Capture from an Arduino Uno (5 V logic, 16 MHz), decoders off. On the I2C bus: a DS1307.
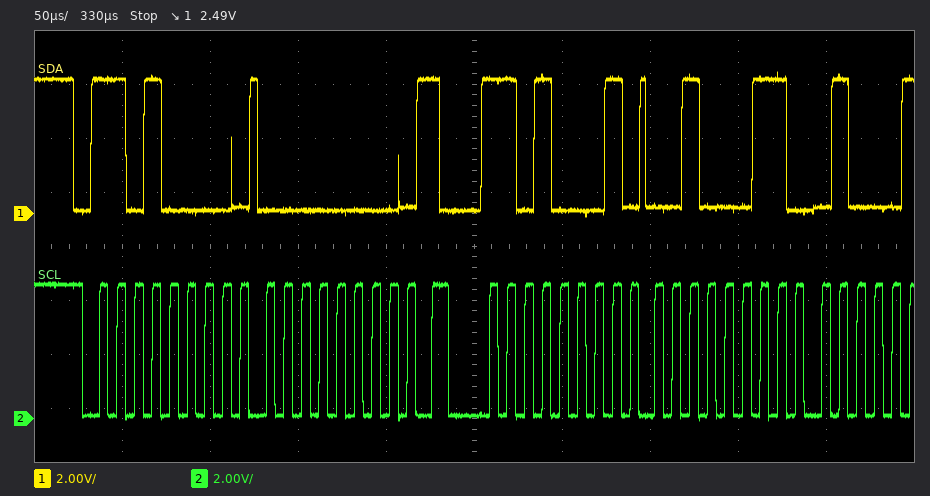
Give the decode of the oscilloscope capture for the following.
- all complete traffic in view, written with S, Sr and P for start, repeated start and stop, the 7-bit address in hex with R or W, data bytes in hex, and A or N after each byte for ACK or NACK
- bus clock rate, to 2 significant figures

S 68W A 00 A Sr 68R A 23 A
100 kHz
